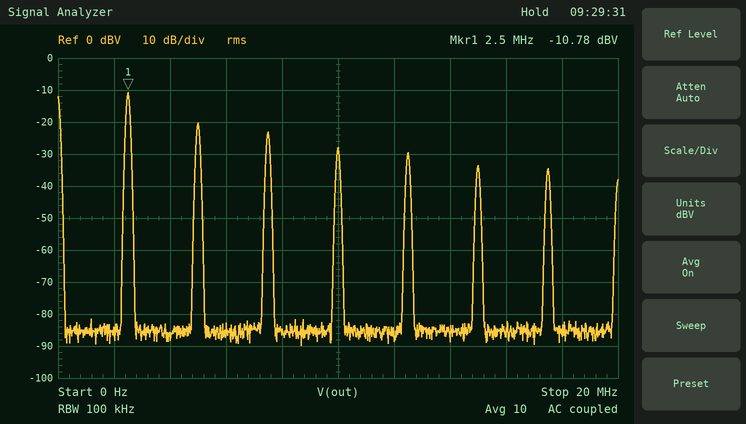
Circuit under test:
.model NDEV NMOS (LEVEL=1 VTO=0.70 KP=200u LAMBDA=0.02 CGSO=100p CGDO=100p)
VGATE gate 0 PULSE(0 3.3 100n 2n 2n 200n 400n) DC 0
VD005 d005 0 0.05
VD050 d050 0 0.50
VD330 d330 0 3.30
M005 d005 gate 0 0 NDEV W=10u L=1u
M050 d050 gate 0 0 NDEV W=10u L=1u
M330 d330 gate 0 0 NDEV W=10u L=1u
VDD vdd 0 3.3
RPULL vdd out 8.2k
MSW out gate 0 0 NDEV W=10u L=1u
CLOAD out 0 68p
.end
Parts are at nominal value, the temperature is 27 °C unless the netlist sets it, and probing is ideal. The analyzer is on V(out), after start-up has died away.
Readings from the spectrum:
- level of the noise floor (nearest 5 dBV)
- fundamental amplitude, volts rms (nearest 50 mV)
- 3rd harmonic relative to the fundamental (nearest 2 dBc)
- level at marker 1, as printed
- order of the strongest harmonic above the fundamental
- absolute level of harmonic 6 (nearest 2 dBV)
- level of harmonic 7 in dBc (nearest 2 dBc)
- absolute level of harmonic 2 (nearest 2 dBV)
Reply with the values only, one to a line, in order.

-85 dBV
300 mV
-12 dBc
-10.78 dBV
2
-34 dBV
-24 dBc
-20 dBV
